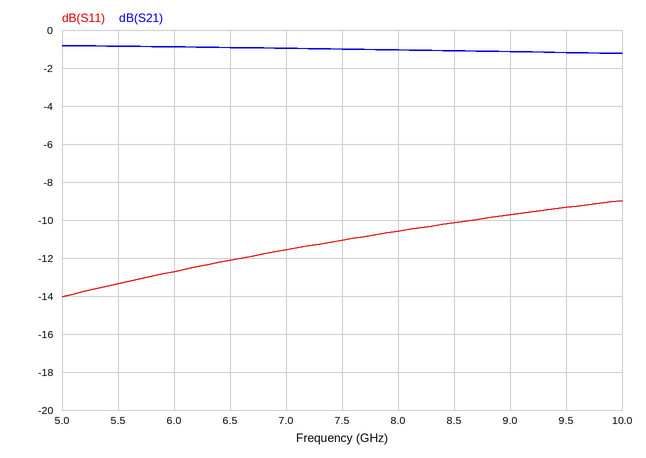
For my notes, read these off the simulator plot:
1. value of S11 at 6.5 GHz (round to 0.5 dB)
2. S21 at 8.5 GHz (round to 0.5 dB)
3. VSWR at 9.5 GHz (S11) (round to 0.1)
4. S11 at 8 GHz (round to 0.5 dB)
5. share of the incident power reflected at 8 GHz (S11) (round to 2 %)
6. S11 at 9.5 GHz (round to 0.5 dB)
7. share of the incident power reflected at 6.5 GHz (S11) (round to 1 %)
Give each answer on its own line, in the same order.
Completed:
-12.0 dB
-1.0 dB
2.0
-10.5 dB
8 %
-9.5 dB
6 %
